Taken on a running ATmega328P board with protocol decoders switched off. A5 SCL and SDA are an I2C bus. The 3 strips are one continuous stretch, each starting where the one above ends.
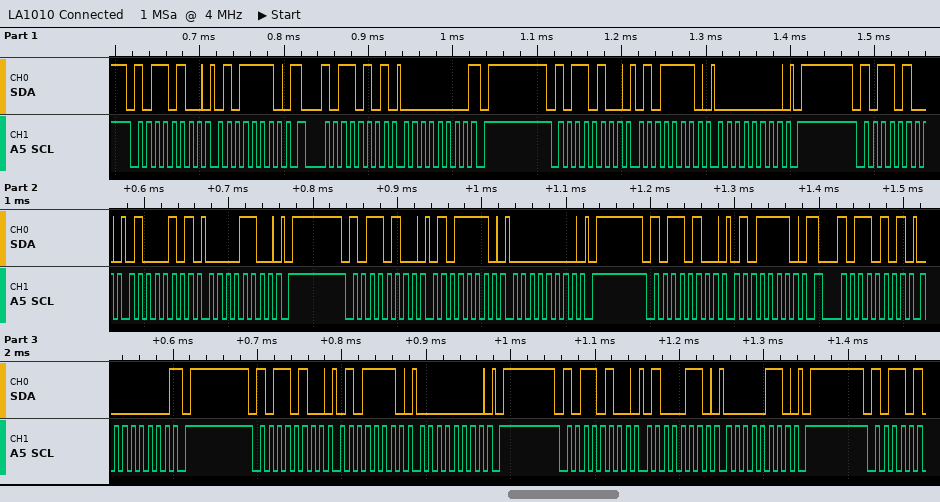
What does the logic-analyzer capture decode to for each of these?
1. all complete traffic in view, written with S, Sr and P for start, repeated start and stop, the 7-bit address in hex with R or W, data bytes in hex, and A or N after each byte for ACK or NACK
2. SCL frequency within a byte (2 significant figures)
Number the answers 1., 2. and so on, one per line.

1. S 5AW A 5E A Sr 5AR A 00 N P S 5AW A 5E A 00 A P S 5AW A 45 A 0C A P S 5AW A 5E A 00 A P S 5AW A 5E A Sr 5AR A 00 N P S 5AW A 5E A 00 A P S 5AW A 46 A 06 A P
2. 100 kHz
